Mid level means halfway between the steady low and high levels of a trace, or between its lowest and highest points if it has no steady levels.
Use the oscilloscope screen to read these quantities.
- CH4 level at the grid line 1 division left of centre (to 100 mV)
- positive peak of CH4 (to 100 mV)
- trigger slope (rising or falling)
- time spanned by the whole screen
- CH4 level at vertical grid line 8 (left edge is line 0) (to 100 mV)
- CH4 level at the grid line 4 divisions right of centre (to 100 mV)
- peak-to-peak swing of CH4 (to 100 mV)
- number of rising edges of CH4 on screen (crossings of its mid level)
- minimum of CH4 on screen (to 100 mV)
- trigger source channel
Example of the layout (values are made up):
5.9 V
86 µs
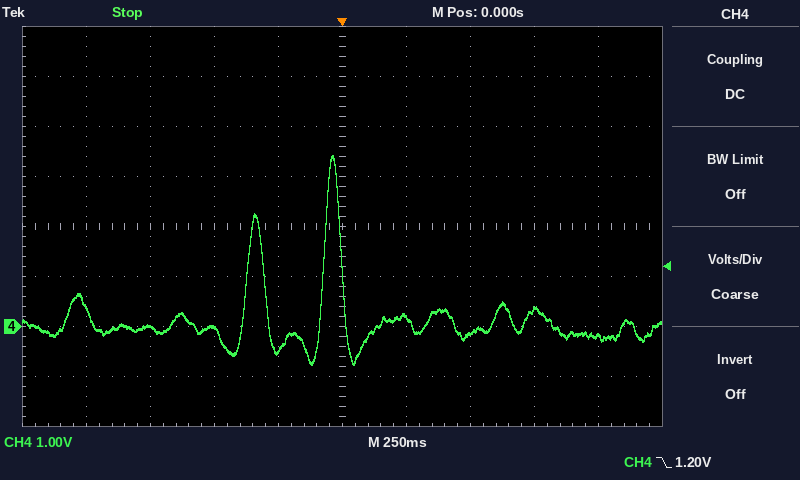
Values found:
-500 mV
3.4 V
falling
2.5 s
300 mV
-200 mV
4.2 V
2
-800 mV
CH4
